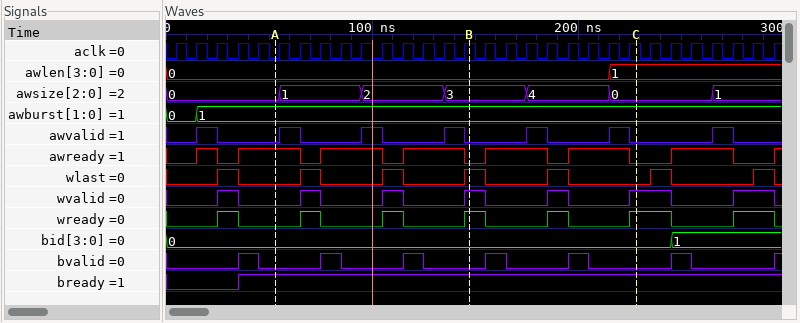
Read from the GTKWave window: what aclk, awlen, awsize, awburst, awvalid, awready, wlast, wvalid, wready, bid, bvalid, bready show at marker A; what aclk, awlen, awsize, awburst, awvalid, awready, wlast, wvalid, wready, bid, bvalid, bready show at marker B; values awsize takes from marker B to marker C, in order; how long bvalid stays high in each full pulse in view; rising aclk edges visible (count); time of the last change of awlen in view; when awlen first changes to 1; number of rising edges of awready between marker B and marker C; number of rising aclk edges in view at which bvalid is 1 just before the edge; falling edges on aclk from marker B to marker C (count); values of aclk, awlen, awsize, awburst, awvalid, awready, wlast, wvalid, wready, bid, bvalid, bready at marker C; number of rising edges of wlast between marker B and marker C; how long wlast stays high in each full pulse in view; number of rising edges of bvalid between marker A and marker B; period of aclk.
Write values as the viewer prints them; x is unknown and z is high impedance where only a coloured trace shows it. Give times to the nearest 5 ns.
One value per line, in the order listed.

aclk=0, awlen=0, awsize=0, awburst=1, awvalid=0, awready=1, wlast=0, wvalid=0, wready=0, bid=0, bvalid=0, bready=1
aclk=1, awlen=0, awsize=3, awburst=1, awvalid=0, awready=0, wlast=1, wvalid=1, wready=1, bid=0, bvalid=0, bready=1
3, 4, 0
10 ns, 10 ns, 10 ns, 10 ns, 10 ns, 10 ns
30
215 ns
215 ns
2
6
8
aclk=1, awlen=1, awsize=0, awburst=1, awvalid=0, awready=0, wlast=0, wvalid=1, wready=1, bid=0, bvalid=0, bready=1
1
10 ns, 10 ns, 10 ns, 10 ns, 10 ns, 10 ns, 10 ns
2
10 ns
